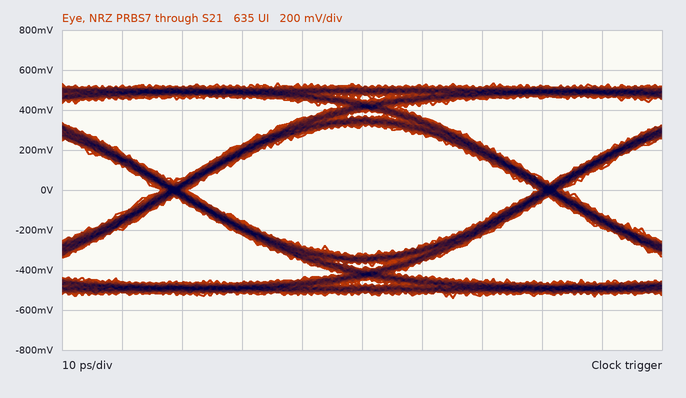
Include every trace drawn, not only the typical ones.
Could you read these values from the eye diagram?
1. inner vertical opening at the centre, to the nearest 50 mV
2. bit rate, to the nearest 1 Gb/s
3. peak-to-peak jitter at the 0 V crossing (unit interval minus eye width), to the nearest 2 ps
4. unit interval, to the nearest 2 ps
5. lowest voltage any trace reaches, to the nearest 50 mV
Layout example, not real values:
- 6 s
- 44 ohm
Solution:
- 650 mV
- 16 Gb/s
- 4 ps
- 62 ps
- -550 mV
